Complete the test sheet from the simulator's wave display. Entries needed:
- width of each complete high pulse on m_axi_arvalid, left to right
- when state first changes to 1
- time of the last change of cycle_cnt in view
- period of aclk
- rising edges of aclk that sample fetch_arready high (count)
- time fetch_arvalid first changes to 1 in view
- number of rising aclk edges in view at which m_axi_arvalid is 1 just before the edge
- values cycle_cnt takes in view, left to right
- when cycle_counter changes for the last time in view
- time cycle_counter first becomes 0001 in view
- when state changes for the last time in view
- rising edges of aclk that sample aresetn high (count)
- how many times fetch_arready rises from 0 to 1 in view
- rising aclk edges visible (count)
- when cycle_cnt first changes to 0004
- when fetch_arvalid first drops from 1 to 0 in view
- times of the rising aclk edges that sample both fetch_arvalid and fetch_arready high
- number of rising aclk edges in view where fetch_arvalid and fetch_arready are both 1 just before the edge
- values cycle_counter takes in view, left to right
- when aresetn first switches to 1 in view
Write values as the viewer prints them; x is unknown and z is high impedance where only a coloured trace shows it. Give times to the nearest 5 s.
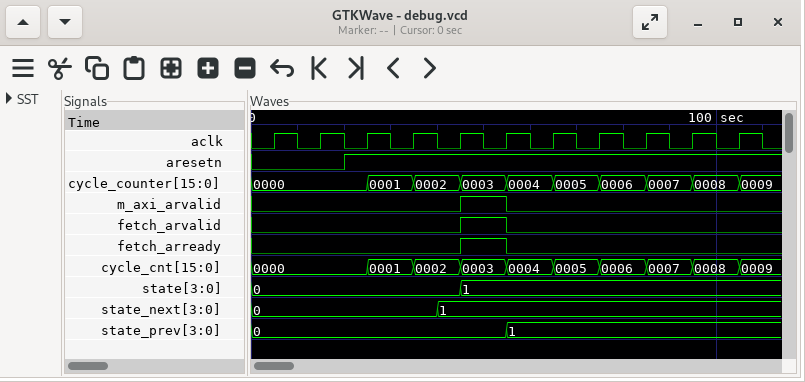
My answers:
10 s
45 s
105 s
10 s
1
45 s
1
0000, 0001, 0002, 0003, 0004, 0005, 0006, 0007, 0008, 0009
105 s
25 s
45 s
9
1
11
55 s
55 s
55 s
1
0000, 0001, 0002, 0003, 0004, 0005, 0006, 0007, 0008, 0009
20 s
